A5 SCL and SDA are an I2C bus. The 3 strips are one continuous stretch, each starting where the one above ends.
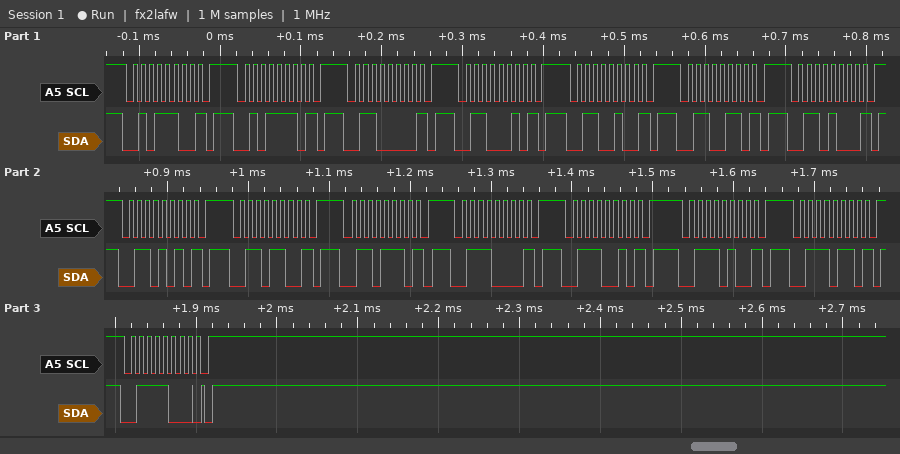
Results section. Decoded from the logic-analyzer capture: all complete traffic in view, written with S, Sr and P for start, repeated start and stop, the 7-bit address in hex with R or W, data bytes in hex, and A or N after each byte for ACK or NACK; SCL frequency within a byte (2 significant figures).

S 2EW N P S 2FW N P S 30W N P S 31W N P S 32W N P S 33W N P S 34W N P S 35W N P S 36W N P S 37W N P S 38W N P S 39W N P S 3AW N P S 3BW N P S 3CW A P
100 kHz
